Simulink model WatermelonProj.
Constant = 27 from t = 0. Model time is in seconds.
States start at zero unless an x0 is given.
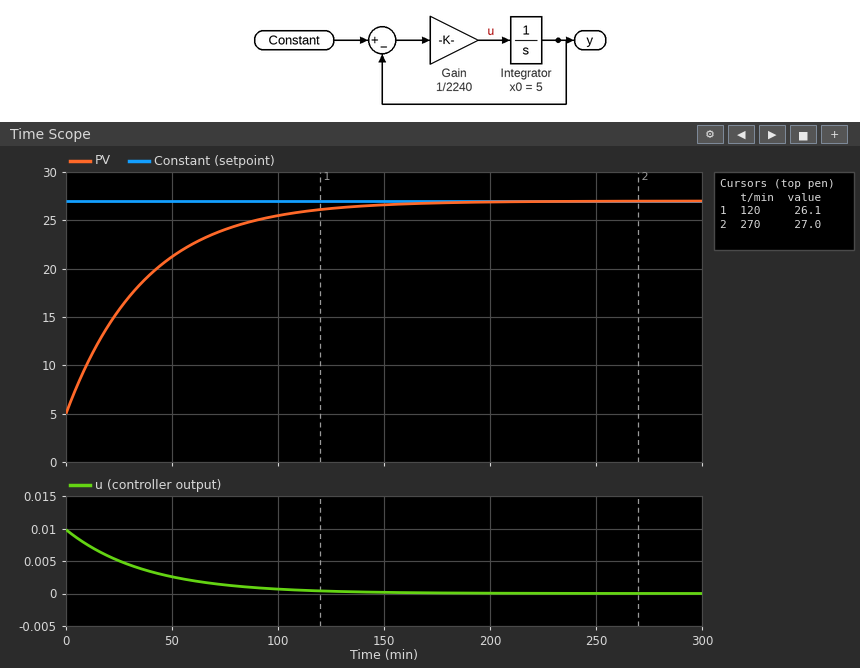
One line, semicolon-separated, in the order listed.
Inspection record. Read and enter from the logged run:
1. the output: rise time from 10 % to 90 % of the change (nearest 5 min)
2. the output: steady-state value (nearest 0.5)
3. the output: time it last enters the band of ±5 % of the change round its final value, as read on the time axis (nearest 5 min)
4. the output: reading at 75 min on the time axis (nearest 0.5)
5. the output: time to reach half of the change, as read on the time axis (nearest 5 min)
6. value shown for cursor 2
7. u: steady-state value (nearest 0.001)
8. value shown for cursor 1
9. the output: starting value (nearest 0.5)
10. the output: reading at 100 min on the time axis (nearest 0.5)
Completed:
80 min; 27.0; 110 min; 24.0; 25 min; 27.0; 0.000; 26.1; 5.0; 25.5
